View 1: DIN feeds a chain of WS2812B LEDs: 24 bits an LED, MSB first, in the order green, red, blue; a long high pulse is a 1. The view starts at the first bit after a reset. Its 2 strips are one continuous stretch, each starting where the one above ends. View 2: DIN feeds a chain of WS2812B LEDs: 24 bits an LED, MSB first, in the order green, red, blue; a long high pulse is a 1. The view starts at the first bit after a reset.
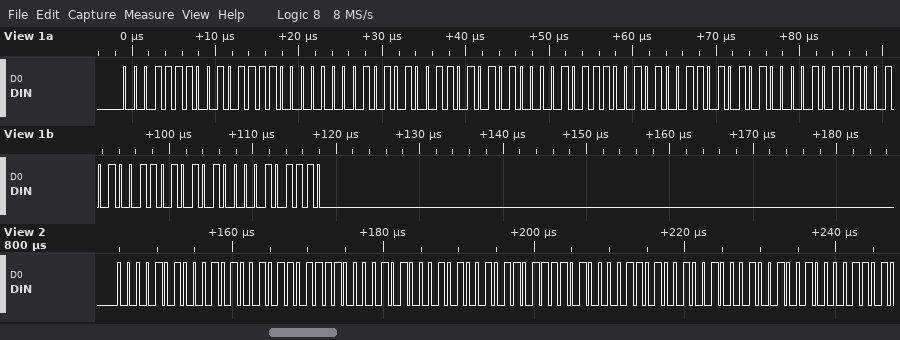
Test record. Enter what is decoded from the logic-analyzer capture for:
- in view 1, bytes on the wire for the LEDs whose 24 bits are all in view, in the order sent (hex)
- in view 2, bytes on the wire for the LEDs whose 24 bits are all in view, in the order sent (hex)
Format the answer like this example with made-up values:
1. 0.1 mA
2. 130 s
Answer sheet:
1. 1E 5E 01 53 54 2E 53 54 2E 53 54 2E
2. 0A 29 6F 0A 29 6F 43 49 12
